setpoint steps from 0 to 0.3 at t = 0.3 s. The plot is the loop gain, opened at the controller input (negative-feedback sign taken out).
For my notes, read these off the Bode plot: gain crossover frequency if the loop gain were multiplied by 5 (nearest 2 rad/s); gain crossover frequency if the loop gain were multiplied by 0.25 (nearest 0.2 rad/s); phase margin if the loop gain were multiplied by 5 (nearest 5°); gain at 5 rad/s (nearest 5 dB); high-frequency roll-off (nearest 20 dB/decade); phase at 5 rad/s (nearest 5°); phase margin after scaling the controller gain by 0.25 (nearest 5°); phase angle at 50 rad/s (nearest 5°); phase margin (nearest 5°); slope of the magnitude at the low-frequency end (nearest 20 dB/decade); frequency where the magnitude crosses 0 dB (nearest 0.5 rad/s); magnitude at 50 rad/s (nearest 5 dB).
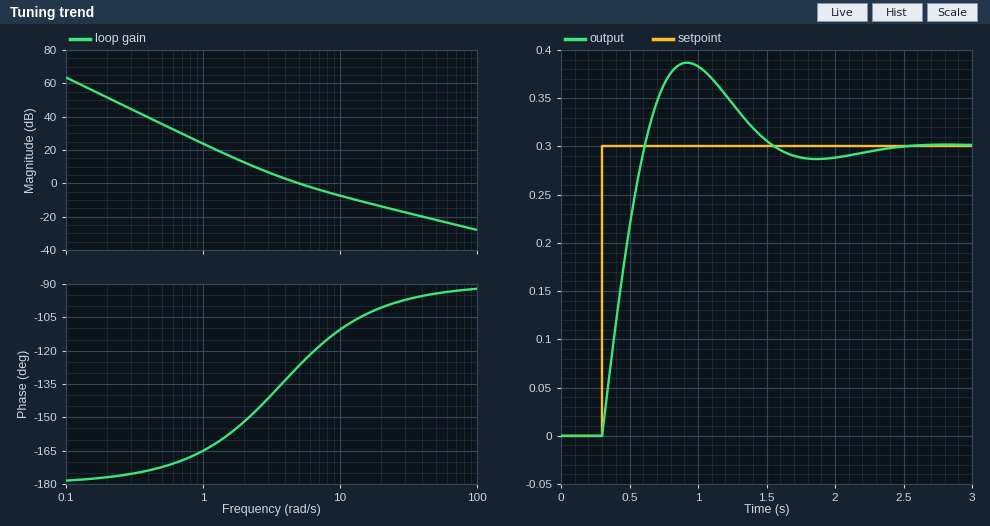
20 rad/s
2.0 rad/s
80°
0 dB
-20 dB/decade
-125°
30°
-95°
55°
-40 dB/decade
5.0 rad/s
-20 dB
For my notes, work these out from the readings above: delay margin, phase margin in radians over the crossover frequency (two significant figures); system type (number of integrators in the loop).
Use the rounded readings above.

0.19 s
2
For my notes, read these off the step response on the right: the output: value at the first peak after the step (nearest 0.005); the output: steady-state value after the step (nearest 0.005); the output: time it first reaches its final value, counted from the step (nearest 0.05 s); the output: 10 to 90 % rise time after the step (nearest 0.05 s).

0.385
0.300
0.30 s
0.25 s
